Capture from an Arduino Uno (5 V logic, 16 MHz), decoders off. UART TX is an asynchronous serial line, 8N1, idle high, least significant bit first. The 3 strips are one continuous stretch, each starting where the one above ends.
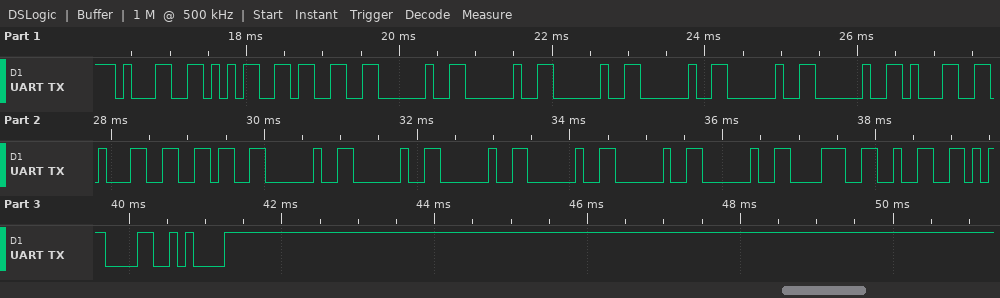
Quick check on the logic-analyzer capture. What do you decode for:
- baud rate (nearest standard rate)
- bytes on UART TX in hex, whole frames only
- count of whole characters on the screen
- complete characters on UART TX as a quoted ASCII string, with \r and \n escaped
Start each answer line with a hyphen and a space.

- 9600 baud
- 0x31 0x35 0x33 0x20 0x20 0x20 0x20 0x20 0x20 0x31 0x31 0x36 0x20 0x20 0x20 0x20 0x20 0x20 0x38 0x32 0x0D 0x0A
- 22
- "153      116      82\r\n"
